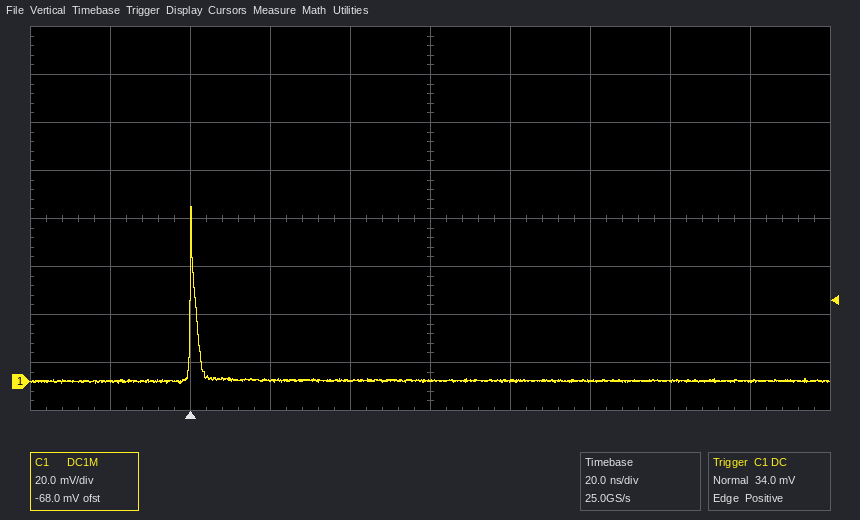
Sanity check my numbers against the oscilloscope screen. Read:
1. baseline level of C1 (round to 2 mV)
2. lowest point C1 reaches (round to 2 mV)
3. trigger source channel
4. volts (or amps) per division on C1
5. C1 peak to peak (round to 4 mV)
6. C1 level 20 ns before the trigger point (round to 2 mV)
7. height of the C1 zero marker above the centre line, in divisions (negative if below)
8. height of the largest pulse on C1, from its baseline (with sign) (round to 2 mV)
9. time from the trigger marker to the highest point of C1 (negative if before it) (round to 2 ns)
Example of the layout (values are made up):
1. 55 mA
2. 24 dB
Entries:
1. 0 mV
2. 0 mV
3. C1
4. 20 mV
5. 72 mV
6. 0 mV
7. -3.4 div
8. +72 mV
9. 0 ns
